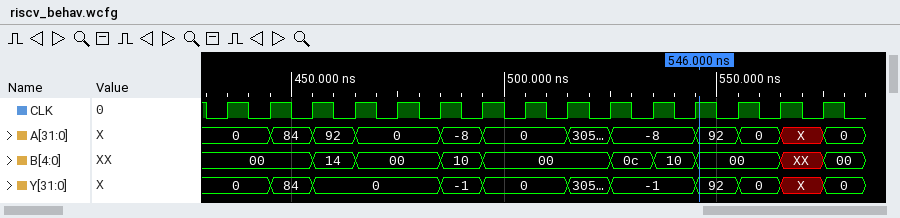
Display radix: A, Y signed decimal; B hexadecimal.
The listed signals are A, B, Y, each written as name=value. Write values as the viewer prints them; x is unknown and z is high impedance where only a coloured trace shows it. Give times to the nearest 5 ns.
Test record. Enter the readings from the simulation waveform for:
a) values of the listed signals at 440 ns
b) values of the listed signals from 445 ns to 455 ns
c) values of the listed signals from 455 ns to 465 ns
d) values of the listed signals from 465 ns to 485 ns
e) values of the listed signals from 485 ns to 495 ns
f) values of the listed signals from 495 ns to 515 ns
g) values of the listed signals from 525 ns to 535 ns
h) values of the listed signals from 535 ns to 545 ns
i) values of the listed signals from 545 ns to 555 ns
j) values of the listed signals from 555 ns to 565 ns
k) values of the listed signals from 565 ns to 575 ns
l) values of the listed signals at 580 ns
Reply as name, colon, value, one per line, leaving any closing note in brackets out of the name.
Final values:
values of the listed signals at 440 ns: A=0, B=00, Y=0
values of the listed signals from 445 ns to 455 ns: A=84, B=00, Y=84
values of the listed signals from 455 ns to 465 ns: A=92, B=14, Y=0
values of the listed signals from 465 ns to 485 ns: A=0, B=00, Y=0
values of the listed signals from 485 ns to 495 ns: A=-8, B=10, Y=-1
values of the listed signals from 495 ns to 515 ns: A=0, B=00, Y=0
values of the listed signals from 525 ns to 535 ns: A=-8, B=0c, Y=-1
values of the listed signals from 535 ns to 545 ns: A=-8, B=10, Y=-1
values of the listed signals from 545 ns to 555 ns: A=92, B=00, Y=92
values of the listed signals from 555 ns to 565 ns: A=0, B=00, Y=0
values of the listed signals from 565 ns to 575 ns: A=X, B=XX, Y=X
values of the listed signals at 580 ns: A=0, B=00, Y=0
